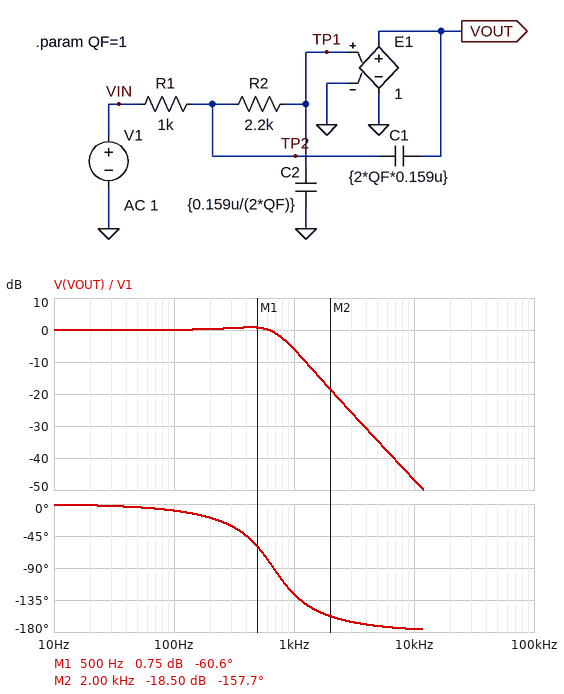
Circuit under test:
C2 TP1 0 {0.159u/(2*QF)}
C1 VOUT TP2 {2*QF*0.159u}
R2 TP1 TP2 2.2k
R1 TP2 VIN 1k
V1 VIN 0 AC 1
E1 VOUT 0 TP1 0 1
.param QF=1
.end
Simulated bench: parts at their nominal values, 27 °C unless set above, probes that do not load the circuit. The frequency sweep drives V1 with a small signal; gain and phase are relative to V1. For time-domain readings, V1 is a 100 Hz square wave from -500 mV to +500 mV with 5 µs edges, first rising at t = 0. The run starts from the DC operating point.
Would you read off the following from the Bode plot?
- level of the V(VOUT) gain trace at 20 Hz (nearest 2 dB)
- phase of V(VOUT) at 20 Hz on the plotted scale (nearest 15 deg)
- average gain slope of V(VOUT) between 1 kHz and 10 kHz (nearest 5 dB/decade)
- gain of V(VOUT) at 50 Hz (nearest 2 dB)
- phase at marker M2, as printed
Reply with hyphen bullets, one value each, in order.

- 0 dB
- 0 deg
- -40 dB/decade
- 0 dB
- -157.7 deg
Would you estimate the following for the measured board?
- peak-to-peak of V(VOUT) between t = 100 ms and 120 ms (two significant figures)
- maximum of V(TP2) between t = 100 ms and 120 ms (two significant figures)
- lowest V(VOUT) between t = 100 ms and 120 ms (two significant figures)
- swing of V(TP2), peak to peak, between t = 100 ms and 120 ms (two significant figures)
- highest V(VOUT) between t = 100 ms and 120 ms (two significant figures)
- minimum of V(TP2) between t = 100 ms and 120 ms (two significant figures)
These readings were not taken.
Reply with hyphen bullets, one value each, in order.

- 1.3 V
- 690 mV
- -630 mV
- 1.4 V
- 630 mV
- -690 mV
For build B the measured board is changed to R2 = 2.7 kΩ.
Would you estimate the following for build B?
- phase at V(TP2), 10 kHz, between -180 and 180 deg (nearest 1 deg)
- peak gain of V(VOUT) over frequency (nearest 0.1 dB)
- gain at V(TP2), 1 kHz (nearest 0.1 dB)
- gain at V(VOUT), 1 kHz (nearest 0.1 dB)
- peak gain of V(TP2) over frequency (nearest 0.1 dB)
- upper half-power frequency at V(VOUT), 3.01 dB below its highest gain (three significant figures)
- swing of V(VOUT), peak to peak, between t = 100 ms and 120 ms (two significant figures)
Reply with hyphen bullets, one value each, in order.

- -90 deg
- 0.6 dB
- -3.5 dB
- -8.0 dB
- 1.8 dB
- 694 Hz
- 1.2 V
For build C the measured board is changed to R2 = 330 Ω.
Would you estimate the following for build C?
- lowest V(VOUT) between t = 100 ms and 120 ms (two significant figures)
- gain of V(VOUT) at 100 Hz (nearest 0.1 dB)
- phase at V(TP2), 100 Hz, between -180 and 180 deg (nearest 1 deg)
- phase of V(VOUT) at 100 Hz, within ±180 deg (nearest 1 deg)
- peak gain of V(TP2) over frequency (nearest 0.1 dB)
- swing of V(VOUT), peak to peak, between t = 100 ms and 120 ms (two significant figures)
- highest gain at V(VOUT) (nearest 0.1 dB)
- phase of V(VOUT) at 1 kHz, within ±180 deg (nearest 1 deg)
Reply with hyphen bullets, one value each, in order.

- -610 mV
- 0 dB
- -3 deg
- -4 deg
- 0.6 dB
- 1.2 V
- 0.5 dB
- -45 deg
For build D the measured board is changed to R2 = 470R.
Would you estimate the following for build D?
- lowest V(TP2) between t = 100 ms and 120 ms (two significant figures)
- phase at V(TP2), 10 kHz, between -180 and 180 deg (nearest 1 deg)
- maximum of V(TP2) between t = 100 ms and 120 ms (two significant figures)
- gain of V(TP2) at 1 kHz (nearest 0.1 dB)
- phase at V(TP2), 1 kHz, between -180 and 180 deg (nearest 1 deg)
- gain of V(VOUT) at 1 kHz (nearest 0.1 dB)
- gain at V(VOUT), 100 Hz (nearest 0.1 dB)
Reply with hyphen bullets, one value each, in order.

- -650 mV
- -104 deg
- 650 mV
- 1.1 dB
- -41 deg
- 0.9 dB
- 0 dB
